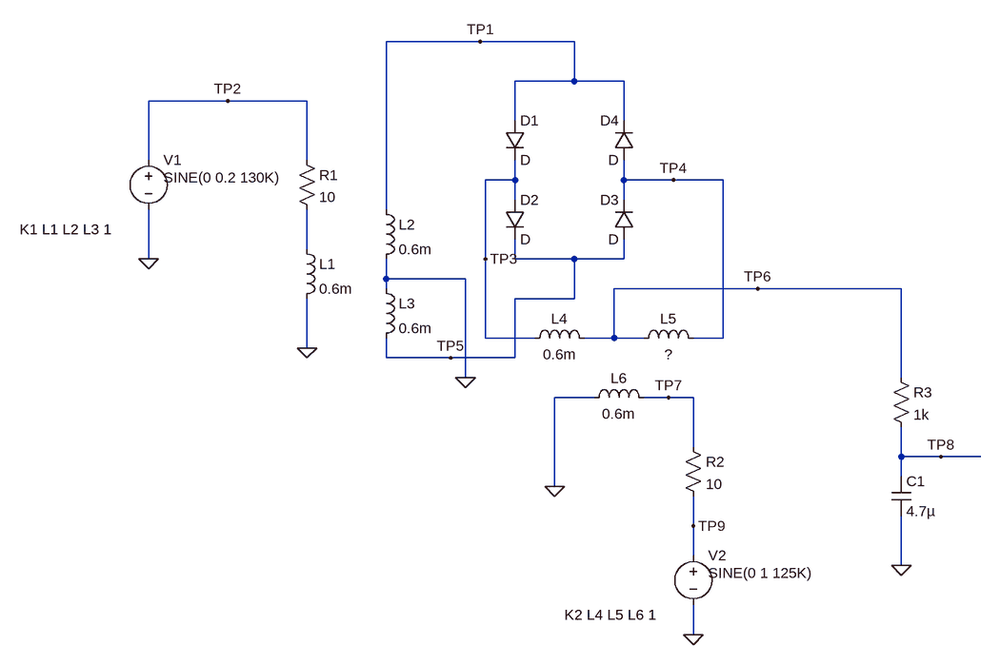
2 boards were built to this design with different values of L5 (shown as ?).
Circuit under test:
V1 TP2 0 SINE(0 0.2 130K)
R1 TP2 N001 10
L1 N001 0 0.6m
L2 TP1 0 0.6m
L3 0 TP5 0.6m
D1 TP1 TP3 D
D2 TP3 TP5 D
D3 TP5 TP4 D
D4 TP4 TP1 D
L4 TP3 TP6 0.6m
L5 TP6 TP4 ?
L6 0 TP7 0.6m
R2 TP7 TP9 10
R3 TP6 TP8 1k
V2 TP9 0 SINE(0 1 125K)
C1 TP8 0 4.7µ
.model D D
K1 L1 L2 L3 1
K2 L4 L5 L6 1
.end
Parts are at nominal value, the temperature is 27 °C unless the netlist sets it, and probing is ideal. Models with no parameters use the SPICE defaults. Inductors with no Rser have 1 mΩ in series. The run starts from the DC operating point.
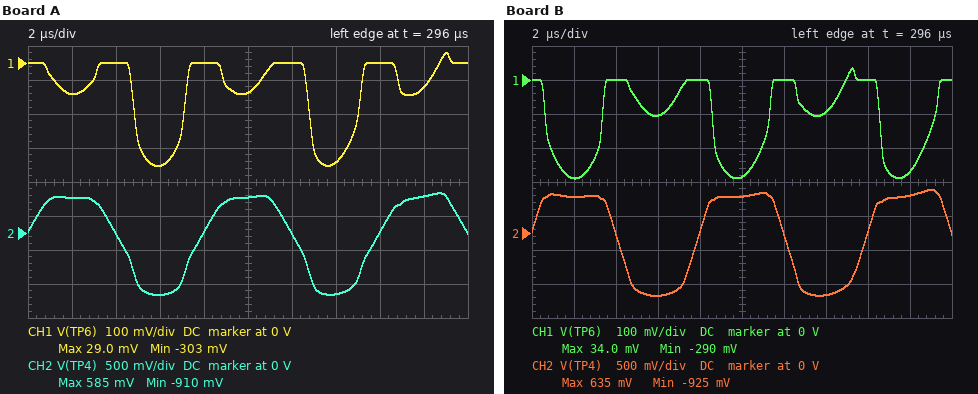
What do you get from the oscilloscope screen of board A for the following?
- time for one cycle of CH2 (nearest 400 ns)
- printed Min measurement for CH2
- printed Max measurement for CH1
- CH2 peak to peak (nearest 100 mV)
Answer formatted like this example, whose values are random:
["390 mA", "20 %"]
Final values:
["8.0 µs", "-910 mV", "29.0 mV", "1.5 V"]
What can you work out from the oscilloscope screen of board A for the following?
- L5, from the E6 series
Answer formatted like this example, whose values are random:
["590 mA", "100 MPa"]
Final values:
["330 µH"]
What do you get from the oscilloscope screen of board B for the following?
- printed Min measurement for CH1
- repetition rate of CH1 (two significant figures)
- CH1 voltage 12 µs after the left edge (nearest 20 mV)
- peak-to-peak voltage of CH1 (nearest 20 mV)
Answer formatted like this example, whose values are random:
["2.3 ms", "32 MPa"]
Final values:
["-290 mV", "130 kHz", "0 V", "320 mV"]
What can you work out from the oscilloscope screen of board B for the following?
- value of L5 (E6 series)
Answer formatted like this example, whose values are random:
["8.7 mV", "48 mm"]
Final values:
["1 mH"]
